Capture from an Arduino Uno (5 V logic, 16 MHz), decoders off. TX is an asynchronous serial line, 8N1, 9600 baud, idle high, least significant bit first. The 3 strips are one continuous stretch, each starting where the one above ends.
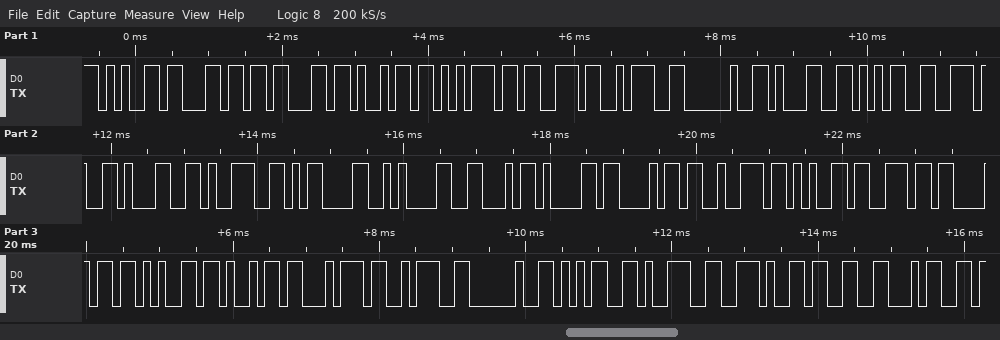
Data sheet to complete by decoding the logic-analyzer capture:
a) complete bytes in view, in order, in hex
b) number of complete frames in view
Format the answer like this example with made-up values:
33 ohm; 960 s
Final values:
65 6C 63 69 75 73 3A 20 31 35 2E 31 39 0D 0A 46 61 68 72 65 6E 68 65 69 74 3A 20 35 39 2E 33 34; 32
